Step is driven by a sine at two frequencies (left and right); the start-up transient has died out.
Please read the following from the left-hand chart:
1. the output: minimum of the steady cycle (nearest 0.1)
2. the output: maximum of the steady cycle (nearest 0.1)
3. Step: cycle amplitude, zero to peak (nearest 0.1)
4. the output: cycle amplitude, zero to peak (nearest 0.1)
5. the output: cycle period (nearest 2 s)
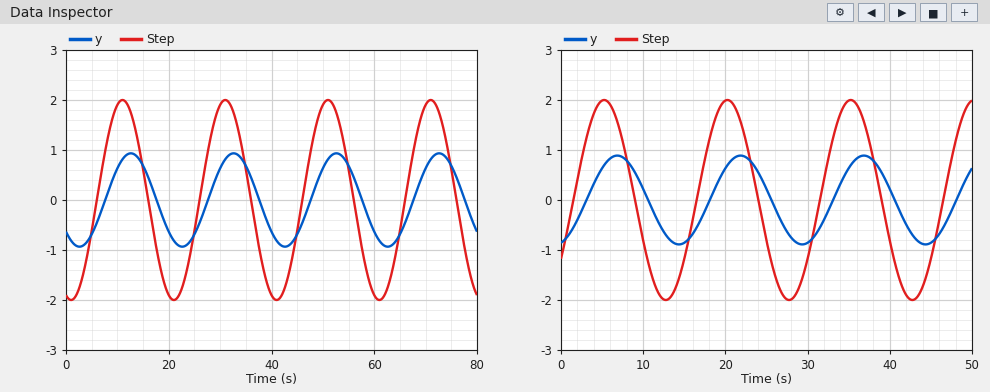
-0.9
0.9
2.0
0.9
20 s
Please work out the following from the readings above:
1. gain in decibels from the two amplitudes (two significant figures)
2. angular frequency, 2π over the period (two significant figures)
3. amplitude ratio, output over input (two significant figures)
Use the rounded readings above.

-6.9 dB
0.31 rad/s
0.45
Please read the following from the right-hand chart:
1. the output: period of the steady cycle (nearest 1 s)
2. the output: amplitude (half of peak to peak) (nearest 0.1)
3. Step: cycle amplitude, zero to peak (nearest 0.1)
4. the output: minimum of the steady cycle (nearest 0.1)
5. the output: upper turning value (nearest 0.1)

15 s
0.9
2.0
-0.9
0.9
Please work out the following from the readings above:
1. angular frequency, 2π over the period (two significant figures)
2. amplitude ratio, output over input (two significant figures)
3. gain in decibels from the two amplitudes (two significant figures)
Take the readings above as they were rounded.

0.42 rad/s
0.45
-6.9 dB
